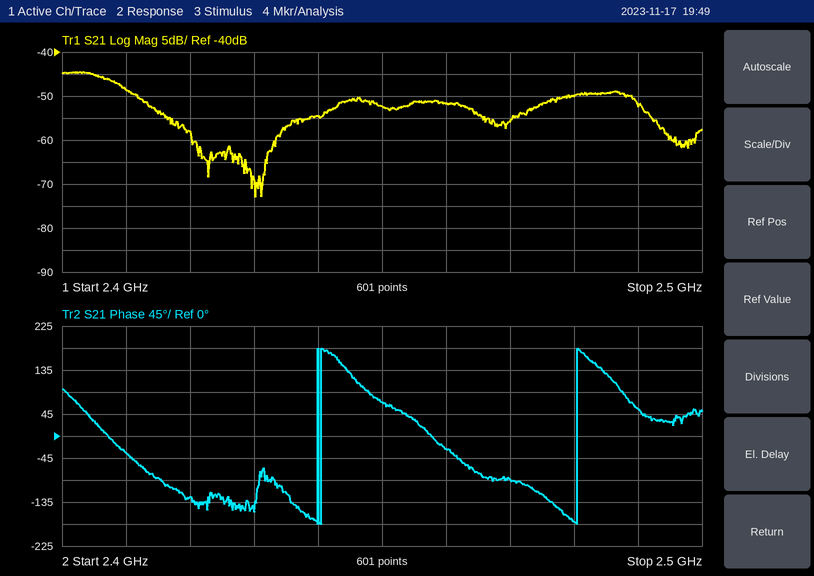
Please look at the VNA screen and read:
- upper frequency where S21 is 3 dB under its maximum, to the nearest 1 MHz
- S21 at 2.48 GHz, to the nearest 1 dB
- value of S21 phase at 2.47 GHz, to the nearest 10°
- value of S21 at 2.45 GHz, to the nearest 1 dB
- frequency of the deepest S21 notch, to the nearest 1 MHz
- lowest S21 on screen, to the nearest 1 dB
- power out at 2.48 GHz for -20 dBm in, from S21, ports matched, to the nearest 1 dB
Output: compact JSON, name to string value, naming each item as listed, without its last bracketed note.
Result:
{"upper frequency where S21 is 3 dB under its maximum, to the nearest 1 MHz": "2.409 GHz", "S21 at 2.48 GHz, to the nearest 1 dB": "-50 dB", "value of S21 phase at 2.47 GHz, to the nearest 10°": "-90°", "value of S21 at 2.45 GHz, to the nearest 1 dB": "-52 dB", "frequency of the deepest S21 notch, to the nearest 1 MHz": "2.430 GHz", "lowest S21 on screen, to the nearest 1 dB": "-73 dB", "power out at 2.48 GHz for -20 dBm in, from S21, ports matched, to the nearest 1 dB": "-70 dBm"}
